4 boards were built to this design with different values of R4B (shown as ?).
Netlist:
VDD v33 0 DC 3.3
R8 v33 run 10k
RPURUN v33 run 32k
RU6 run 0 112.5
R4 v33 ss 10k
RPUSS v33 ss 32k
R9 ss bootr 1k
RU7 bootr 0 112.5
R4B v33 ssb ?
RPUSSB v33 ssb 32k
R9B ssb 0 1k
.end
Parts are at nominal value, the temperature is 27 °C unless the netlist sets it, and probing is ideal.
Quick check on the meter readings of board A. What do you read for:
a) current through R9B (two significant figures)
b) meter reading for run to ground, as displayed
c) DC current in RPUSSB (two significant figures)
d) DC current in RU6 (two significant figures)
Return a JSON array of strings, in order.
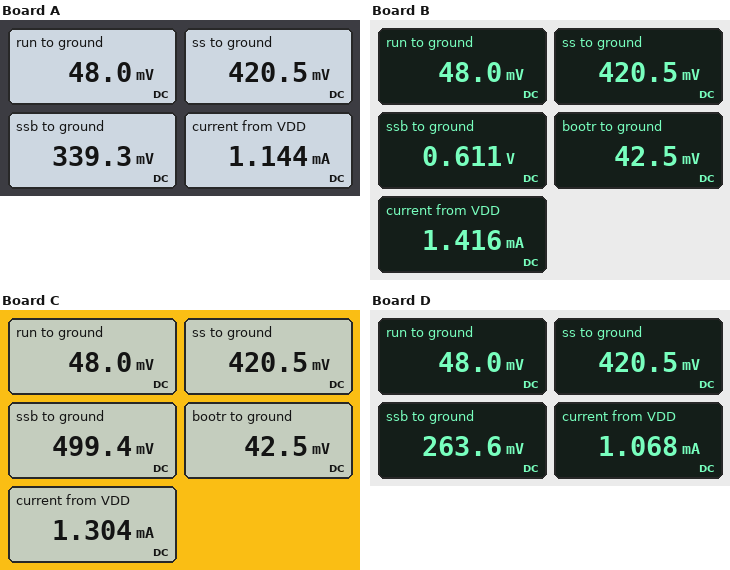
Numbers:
["340 µA", "48.0 mV", "93 µA", "430 µA"]
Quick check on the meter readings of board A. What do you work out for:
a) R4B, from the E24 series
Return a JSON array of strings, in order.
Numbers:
["12 kΩ"]
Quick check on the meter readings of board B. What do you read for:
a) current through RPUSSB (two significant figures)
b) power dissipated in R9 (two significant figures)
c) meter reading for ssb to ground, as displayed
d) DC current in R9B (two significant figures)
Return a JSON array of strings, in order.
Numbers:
["84 µA", "140 µW", "0.611 V", "610 µA"]
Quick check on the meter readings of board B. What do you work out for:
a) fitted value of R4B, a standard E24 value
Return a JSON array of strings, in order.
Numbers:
["5.1 kΩ"]
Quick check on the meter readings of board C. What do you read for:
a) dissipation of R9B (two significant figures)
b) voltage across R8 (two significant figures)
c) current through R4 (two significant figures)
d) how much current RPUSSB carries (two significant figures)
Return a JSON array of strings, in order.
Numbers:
["250 µW", "3.3 V", "290 µA", "88 µA"]
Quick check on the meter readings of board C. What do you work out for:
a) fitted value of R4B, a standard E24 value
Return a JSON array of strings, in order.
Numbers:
["6.8 kΩ"]
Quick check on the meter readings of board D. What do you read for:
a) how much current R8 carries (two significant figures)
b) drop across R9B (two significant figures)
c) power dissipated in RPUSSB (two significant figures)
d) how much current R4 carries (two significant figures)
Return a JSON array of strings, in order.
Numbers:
["330 µA", "260 mV", "290 µW", "290 µA"]
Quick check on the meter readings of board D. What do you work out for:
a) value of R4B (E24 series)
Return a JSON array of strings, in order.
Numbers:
["18 kΩ"]
